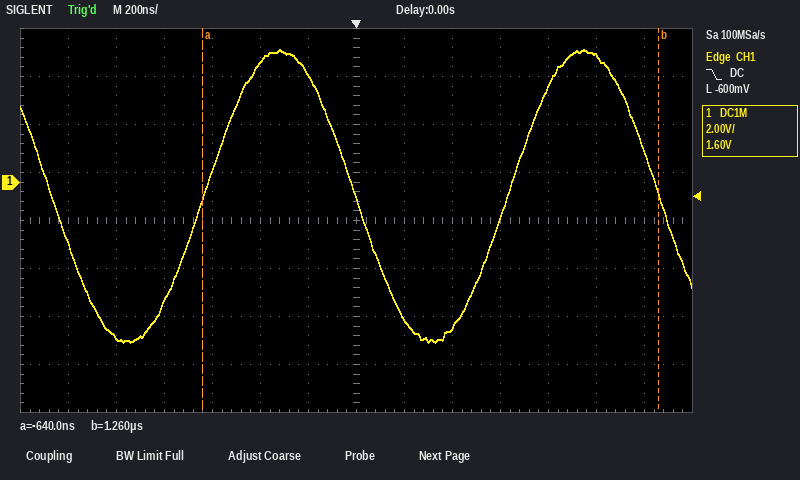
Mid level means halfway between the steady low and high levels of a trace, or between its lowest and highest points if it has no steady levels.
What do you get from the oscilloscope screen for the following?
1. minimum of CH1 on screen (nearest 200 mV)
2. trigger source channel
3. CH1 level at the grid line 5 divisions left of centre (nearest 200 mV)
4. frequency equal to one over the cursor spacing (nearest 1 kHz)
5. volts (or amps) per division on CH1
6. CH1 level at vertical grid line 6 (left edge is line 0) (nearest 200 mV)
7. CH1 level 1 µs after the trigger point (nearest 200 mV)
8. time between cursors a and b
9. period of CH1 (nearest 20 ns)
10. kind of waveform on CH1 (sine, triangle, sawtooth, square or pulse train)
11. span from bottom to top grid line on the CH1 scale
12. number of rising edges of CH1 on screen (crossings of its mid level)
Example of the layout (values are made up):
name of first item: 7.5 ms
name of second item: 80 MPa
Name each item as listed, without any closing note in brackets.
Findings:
minimum of CH1 on screen: -6.6 V
trigger source channel: CH1
CH1 level at the grid line 5 divisions left of centre: -6.4 V
frequency equal to one over the cursor spacing: 526 kHz
volts (or amps) per division on CH1: 2 V
CH1 level at vertical grid line 6 (left edge is line 0): 4.4 V
CH1 level 1 µs after the trigger point: 5.2 V
time between cursors a and b: 1.90 µs
period of CH1: 1.26 µs
kind of waveform on CH1: sine
span from bottom to top grid line on the CH1 scale: 16 V
number of rising edges of CH1 on screen: 2
